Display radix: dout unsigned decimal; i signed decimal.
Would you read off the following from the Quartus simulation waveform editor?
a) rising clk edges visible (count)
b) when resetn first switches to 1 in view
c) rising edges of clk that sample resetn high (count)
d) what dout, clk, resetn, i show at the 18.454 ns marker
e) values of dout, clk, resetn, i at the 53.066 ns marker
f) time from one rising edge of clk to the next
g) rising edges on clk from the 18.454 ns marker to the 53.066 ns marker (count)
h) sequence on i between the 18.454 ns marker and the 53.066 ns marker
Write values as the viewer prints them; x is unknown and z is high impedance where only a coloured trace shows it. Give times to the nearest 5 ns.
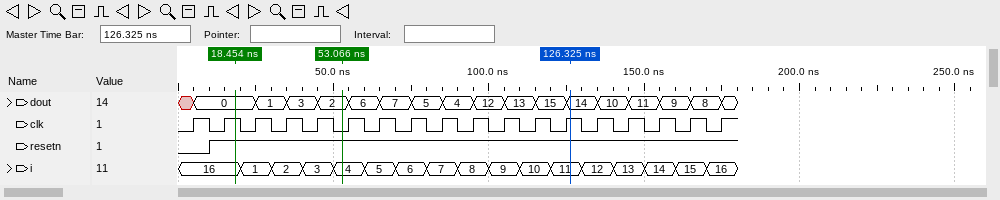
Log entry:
18
10 ns
17
dout=0, clk=1, resetn=1, i=16
dout=2, clk=0, resetn=1, i=4
10 ns
3
16, 1, 2, 3, 4
